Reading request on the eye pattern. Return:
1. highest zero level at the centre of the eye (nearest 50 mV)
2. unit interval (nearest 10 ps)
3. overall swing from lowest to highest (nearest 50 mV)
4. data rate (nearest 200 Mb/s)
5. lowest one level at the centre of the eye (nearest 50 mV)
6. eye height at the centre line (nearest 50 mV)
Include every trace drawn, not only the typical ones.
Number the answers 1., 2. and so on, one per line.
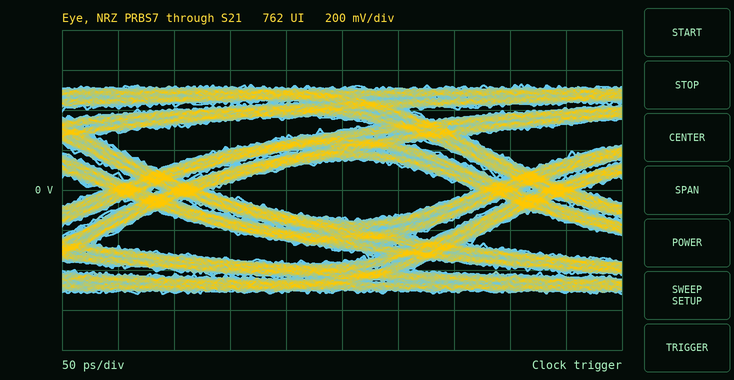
1. -150 mV
2. 330 ps
3. 1.05 V
4. 3.0 Gb/s
5. 150 mV
6. 300 mV
